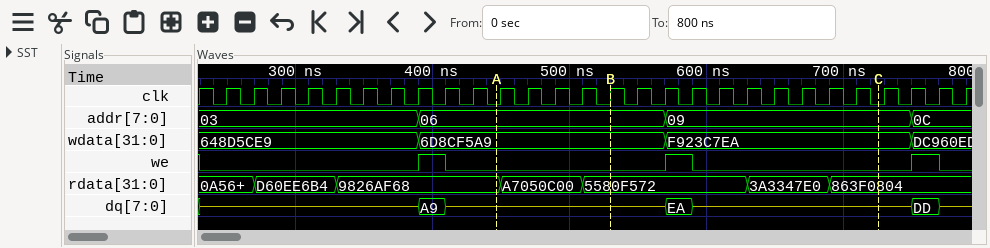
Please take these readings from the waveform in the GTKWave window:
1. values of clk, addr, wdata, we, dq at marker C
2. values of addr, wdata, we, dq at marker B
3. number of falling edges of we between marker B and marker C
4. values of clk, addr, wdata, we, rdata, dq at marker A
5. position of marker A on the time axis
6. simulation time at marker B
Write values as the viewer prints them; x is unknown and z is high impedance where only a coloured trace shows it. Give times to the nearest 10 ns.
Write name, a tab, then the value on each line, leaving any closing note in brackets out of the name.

values of clk, addr, wdata, we, dq at marker C	clk=0, addr=09, wdata=F923C7EA, we=0, dq=z
values of addr, wdata, we, dq at marker B	addr=06, wdata=6D8CF5A9, we=0, dq=z
number of falling edges of we between marker B and marker C	1
values of clk, addr, wdata, we, rdata, dq at marker A	clk=0, addr=06, wdata=6D8CF5A9, we=0, rdata=9826AF68, dq=z
position of marker A on the time axis	450 ns
simulation time at marker B	530 ns
